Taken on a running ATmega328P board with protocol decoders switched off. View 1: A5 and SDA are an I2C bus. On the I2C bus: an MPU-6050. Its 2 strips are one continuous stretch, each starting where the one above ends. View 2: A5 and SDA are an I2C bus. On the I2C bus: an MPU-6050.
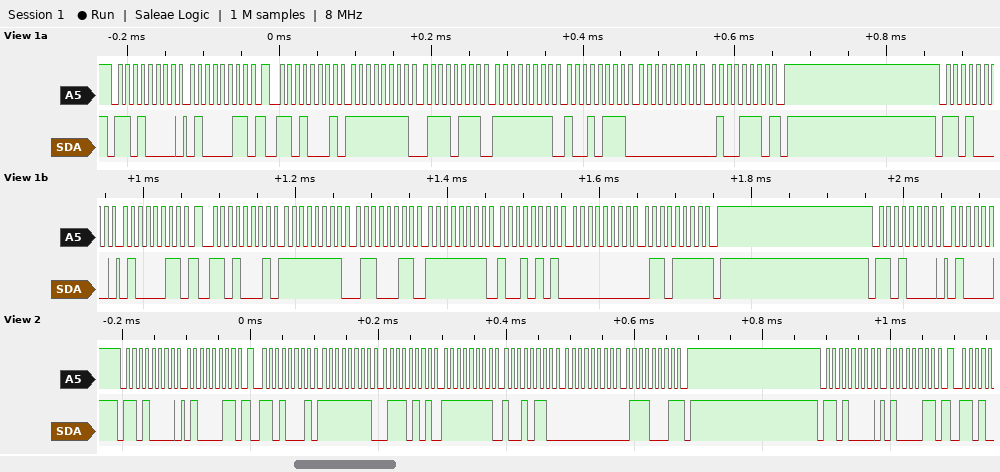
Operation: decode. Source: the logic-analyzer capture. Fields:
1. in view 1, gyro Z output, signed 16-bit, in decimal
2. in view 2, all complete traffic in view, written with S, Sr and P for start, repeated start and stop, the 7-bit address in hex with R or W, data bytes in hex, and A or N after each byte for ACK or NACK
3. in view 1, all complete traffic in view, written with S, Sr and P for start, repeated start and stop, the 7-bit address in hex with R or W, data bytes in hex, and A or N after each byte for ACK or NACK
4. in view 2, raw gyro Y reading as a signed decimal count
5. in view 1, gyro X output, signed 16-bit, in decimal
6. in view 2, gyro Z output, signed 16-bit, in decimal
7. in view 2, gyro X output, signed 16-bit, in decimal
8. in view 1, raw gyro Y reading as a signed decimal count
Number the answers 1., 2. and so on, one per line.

1. 78
2. S 68W A 43 A Sr 68R A FF A 75 A FF A 96 A 00 A 71 N P S 68W A 43 A
3. S 68W A 43 A Sr 68R A FF A 77 A FF A 97 A 00 A 4E N P S 68W A 43 A Sr 68R A FF A 63 A FF A 95 A 00 A 6F N P S 68W A
4. -106
5. -137
6. 113
7. -139
8. -105
